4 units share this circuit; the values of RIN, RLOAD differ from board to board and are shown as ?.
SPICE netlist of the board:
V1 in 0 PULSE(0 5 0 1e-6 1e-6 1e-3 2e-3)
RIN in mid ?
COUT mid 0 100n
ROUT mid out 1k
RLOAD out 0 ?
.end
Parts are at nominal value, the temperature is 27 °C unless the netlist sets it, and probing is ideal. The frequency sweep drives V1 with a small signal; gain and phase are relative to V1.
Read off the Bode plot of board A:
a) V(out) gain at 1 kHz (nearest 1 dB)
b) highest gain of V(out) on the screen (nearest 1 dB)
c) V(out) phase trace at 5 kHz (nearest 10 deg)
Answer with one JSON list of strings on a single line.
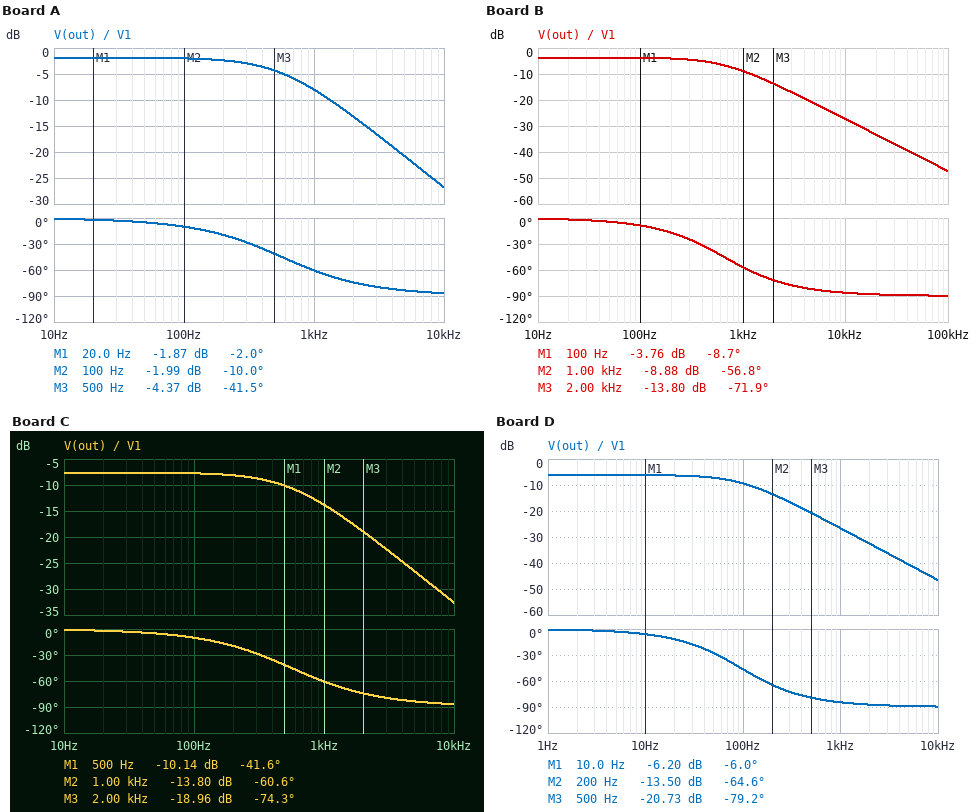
["-8 dB", "-2 dB", "-80 deg"]
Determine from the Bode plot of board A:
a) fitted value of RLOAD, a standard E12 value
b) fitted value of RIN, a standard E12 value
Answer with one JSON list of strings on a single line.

["18 kΩ", "3.3 kΩ"]
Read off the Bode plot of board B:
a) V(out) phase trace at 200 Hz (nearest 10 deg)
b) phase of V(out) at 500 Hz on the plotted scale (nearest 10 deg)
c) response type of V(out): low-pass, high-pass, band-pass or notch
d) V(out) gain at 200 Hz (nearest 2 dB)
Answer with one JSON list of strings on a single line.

["-20 deg", "-40 deg", "low-pass", "-4 dB"]
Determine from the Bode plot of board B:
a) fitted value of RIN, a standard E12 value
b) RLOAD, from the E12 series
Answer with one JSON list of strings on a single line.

["3.3 kΩ", "8.2 kΩ"]
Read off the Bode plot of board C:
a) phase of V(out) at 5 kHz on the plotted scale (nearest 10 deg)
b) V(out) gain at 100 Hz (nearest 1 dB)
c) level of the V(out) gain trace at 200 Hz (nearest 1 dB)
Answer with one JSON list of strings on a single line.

["-80 deg", "-8 dB", "-8 dB"]
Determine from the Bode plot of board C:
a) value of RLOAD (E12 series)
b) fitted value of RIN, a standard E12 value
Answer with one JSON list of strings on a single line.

["4.7 kΩ", "5.6 kΩ"]
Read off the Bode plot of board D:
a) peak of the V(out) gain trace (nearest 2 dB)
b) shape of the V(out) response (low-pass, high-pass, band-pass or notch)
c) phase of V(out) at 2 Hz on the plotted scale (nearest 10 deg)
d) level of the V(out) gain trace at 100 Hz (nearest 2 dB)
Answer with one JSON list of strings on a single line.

["-6 dB", "low-pass", "0 deg", "-10 dB"]
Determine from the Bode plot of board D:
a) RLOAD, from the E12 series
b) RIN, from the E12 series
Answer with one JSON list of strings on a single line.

["33 kΩ", "33 kΩ"]
